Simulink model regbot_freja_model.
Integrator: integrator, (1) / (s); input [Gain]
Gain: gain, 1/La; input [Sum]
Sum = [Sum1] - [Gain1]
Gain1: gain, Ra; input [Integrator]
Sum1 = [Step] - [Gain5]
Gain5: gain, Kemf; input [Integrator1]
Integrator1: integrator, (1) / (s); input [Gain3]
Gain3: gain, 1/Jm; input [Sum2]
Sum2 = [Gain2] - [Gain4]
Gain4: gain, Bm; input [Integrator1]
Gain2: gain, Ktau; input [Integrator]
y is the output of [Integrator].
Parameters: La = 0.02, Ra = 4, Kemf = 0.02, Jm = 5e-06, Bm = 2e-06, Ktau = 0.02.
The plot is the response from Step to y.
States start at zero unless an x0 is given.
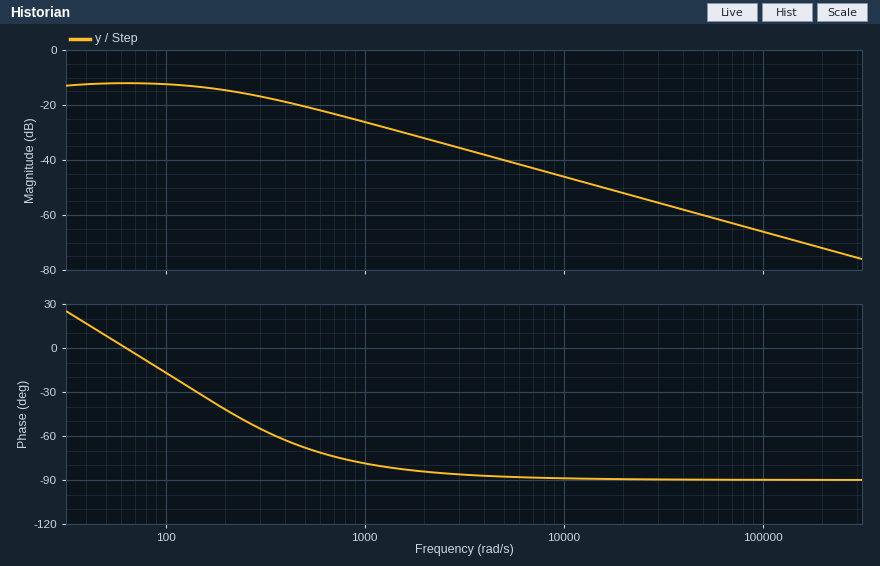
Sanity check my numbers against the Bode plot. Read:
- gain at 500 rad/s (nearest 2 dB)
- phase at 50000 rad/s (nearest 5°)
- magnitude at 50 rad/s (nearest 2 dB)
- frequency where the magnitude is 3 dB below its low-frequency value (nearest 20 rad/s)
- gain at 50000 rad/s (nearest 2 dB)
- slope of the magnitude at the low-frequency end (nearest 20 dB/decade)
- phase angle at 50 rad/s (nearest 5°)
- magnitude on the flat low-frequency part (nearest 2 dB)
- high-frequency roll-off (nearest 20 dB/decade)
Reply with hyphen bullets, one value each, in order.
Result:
- -20 dB
- -90°
- -12 dB
- 220 rad/s
- -60 dB
- 0 dB/decade
- 10°
- -12 dB
- -20 dB/decade
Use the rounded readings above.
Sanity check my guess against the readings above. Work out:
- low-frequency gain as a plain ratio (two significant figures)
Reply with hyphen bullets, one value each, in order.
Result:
- 0.25
